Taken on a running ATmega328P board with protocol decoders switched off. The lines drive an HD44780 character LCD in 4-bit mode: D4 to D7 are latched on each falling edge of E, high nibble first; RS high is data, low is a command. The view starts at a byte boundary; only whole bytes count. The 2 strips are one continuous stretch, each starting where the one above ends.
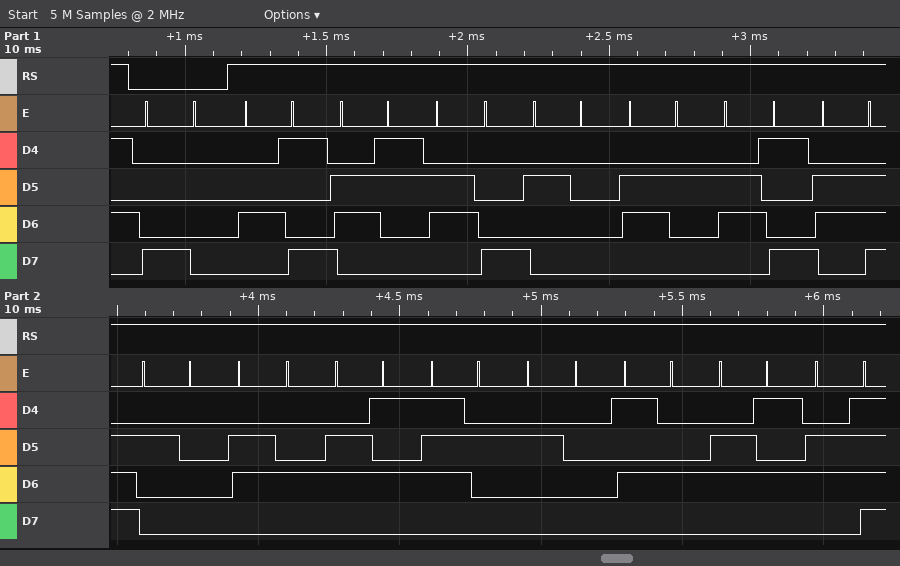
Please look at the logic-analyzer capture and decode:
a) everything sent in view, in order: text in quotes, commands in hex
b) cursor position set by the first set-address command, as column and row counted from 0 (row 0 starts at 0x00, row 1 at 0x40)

0x80 "Ich bin der Teo"
column 0, row 0
